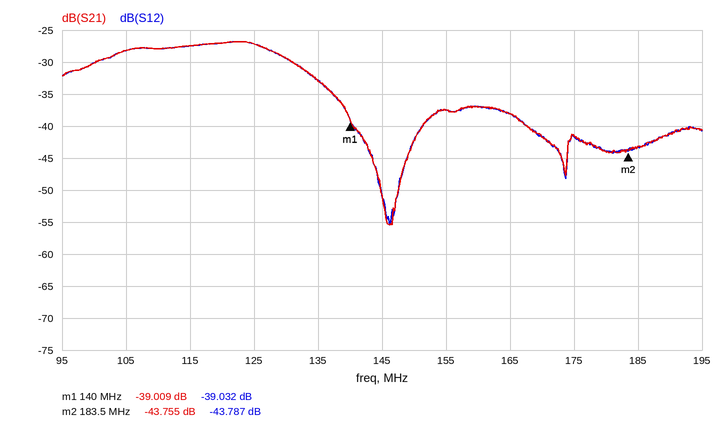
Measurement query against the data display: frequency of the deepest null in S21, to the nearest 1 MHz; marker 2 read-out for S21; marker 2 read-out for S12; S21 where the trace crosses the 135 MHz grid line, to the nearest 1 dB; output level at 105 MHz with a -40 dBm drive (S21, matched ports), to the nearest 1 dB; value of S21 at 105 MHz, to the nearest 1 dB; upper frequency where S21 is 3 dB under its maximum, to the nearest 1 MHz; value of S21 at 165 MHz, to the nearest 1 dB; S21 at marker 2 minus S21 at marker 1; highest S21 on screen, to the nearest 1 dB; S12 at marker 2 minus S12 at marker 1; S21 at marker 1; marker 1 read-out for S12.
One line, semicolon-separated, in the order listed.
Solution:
146 MHz; -43.755 dB; -43.787 dB; -33 dB; -68 dBm; -28 dB; 131 MHz; -38 dB; -4.746 dB; -27 dB; -4.755 dB; -39.009 dB; -39.032 dB
